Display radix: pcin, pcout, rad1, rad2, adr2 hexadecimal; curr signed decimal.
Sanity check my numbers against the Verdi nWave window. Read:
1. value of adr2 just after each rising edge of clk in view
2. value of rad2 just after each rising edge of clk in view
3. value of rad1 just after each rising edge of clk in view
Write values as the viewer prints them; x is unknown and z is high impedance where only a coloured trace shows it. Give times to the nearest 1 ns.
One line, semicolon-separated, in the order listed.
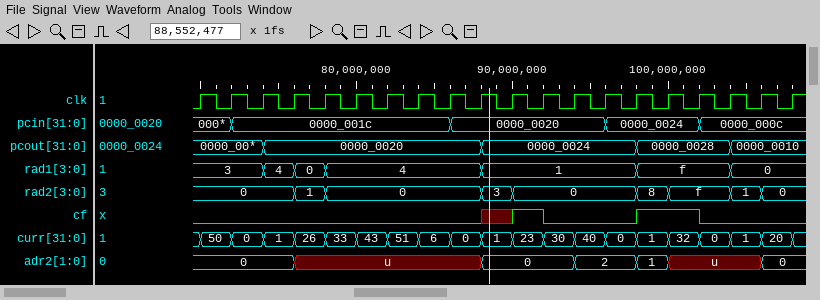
0, 0, 0, u, u, u, u, u, u, 0, 0, 0, 2, 2, 1, u, u, u, 0, 0; 0, 0, 0, 1, 0, 0, 0, 0, 0, 3, 0, 0, 0, 0, 8, f, f, 1, 0, 0; 3, 3, 4, 0, 4, 4, 4, 4, 4, 1, 1, 1, 1, 1, f, f, f, 0, 0, 0
